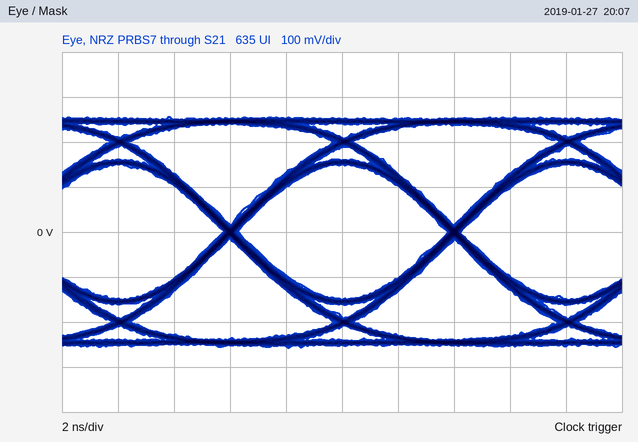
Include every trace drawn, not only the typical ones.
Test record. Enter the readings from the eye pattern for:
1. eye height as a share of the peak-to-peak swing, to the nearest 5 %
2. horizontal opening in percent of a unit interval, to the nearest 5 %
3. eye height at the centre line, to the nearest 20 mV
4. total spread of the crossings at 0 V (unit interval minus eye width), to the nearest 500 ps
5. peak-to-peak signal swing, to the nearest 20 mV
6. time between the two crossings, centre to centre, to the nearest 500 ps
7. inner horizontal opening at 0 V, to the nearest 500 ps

60 %
95 %
300 mV
500 ps
520 mV
8.0 ns
7.5 ns
